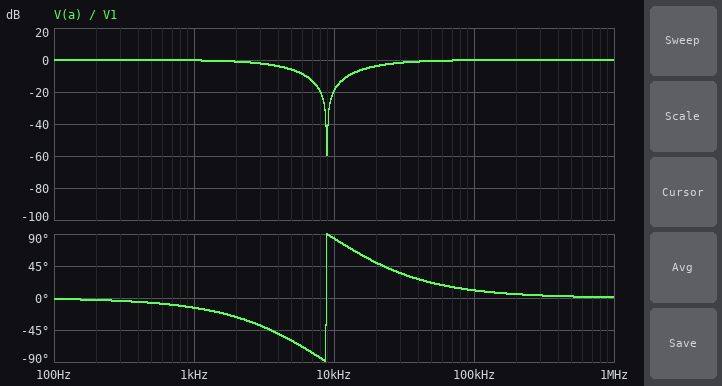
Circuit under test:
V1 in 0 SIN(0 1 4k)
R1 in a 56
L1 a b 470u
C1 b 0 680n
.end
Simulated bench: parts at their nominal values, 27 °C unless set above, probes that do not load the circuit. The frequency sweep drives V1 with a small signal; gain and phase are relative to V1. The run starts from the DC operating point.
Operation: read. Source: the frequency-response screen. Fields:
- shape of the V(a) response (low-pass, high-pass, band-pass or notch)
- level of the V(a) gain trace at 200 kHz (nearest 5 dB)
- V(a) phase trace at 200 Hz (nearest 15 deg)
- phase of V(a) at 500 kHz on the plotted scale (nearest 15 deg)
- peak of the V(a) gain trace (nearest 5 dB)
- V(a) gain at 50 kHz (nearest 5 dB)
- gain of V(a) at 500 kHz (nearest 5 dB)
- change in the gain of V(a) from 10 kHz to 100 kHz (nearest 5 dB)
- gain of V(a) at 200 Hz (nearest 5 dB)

notch
0 dB
0 deg
0 deg
0 dB
0 dB
0 dB
20 dB
0 dB
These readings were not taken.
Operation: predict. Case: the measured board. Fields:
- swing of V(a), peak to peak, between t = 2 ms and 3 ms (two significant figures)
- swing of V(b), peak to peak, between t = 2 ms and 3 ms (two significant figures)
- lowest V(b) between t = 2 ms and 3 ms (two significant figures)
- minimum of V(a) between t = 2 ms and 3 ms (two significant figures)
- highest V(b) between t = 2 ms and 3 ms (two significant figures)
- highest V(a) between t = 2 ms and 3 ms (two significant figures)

1.3 V
1.6 V
-800 mV
-640 mV
800 mV
640 mV
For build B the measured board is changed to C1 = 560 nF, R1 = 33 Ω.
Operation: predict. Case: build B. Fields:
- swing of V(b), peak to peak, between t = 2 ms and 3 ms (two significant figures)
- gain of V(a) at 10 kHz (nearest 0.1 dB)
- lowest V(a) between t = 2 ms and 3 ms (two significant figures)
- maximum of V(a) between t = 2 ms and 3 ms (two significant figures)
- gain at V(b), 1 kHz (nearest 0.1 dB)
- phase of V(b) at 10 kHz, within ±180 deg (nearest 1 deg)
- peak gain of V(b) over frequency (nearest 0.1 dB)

2.1 V
-29.5 dB
-870 mV
870 mV
0 dB
-92 deg
0.6 dB
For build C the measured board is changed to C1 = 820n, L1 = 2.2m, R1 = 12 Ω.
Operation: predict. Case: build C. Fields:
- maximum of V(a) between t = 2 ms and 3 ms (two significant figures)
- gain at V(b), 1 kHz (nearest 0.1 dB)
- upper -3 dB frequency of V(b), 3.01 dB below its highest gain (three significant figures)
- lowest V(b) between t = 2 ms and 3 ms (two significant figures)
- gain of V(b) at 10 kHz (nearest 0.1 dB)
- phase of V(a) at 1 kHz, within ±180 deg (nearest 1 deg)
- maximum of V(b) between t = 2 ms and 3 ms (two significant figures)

490 mV
0.6 dB
4.11 kHz
-3.5 V
-15.8 dB
-4 deg
3.5 V
